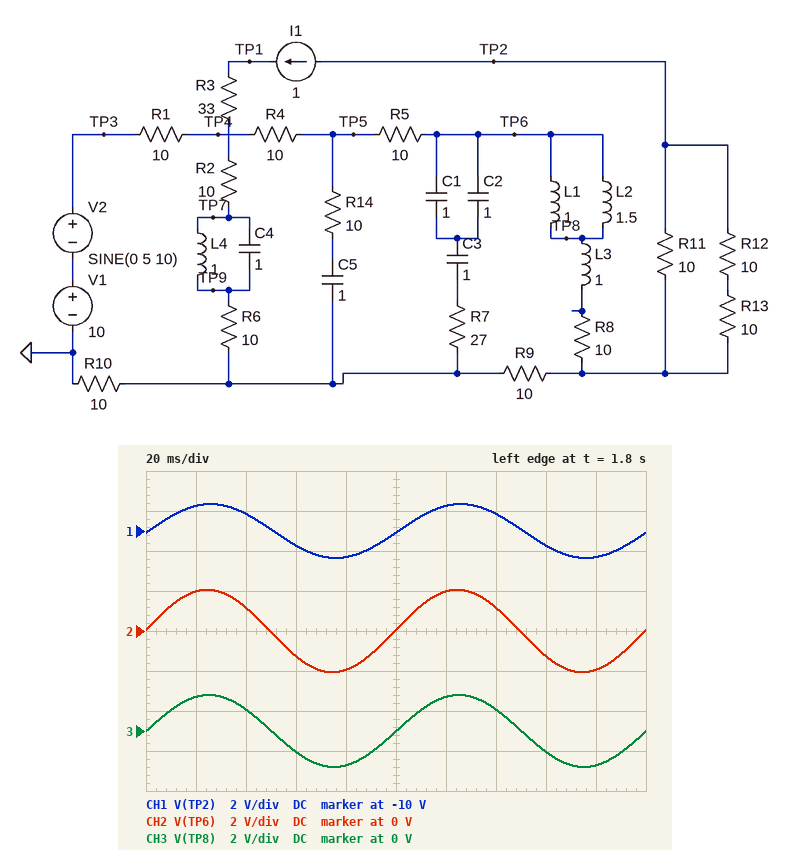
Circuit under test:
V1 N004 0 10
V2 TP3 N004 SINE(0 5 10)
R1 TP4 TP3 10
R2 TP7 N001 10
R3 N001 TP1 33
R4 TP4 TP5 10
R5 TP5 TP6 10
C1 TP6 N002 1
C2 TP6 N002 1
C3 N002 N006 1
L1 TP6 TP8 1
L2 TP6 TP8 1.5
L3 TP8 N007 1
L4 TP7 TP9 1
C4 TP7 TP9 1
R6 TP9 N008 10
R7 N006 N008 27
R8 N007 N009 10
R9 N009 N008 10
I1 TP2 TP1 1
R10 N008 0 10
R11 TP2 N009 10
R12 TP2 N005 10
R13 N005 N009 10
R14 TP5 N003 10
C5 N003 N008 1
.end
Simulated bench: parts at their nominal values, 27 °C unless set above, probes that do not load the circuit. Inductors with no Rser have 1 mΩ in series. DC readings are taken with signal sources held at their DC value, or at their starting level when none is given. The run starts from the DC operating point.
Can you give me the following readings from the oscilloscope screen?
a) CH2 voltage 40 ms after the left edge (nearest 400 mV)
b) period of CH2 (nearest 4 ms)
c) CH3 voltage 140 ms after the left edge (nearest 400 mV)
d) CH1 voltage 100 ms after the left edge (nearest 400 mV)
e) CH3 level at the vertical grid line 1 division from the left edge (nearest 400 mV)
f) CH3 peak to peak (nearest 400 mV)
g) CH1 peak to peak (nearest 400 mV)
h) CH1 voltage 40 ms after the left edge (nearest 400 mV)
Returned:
1.2 V
100 ms
1.2 V
-10.0 V
1.6 V
3.6 V
2.8 V
-9.2 V
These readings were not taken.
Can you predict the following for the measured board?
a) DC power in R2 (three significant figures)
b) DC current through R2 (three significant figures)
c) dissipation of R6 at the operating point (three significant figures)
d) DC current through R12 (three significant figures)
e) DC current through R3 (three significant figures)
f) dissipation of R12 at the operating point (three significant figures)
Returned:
10.0 W
1.00 A
10.0 W
333 mA
1.00 A
1.11 W
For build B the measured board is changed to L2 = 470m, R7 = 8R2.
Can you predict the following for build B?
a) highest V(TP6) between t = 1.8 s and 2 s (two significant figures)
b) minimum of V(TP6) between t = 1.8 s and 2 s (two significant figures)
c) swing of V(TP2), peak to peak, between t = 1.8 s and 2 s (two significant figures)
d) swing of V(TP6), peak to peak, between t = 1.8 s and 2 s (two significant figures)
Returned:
1.8 V
-1.8 V
2.8 V
3.5 V
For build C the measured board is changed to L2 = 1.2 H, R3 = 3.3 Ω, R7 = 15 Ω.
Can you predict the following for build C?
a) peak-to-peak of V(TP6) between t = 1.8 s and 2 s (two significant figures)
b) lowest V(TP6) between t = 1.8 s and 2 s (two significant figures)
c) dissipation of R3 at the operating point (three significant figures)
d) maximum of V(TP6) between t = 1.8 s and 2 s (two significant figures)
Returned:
3.8 V
-1.9 V
3.30 W
1.9 V
